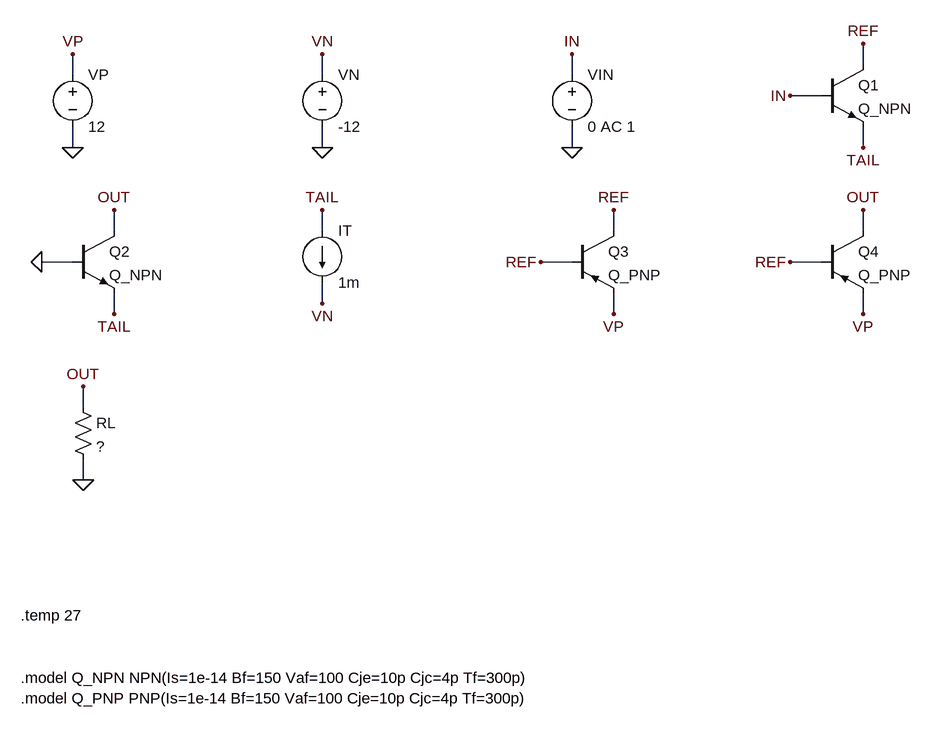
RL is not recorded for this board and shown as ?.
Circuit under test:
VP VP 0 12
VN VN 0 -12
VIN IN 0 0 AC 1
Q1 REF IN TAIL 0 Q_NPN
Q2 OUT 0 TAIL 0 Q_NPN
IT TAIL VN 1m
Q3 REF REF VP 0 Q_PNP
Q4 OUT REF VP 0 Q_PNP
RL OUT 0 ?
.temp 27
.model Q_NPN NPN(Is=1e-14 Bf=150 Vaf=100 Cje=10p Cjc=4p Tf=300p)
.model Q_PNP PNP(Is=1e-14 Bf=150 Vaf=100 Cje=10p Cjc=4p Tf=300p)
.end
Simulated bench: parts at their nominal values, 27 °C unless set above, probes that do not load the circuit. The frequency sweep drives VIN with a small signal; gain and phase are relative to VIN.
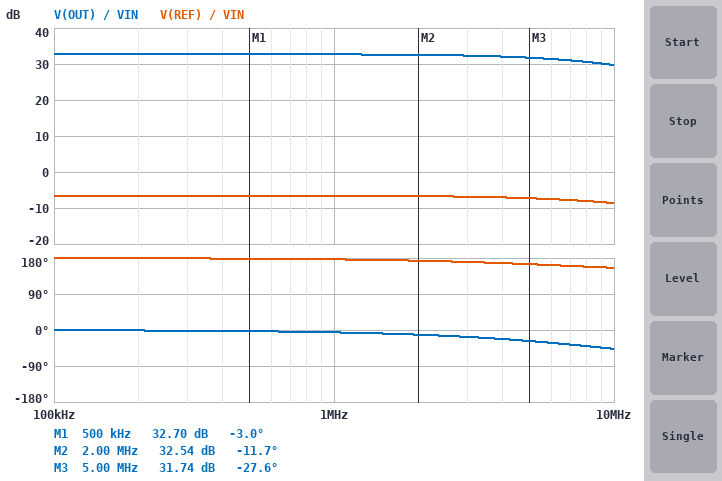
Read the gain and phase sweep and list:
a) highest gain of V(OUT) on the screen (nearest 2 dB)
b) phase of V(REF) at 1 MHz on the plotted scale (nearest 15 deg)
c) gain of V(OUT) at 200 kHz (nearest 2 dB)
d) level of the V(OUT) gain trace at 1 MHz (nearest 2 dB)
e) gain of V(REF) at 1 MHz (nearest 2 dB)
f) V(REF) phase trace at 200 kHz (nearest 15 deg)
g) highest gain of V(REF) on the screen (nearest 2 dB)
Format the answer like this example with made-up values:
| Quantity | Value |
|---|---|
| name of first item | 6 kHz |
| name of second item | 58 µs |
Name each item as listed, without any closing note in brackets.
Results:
| Quantity | Value |
|---|---|
| highest gain of V(OUT) on the screen | 32 dB |
| phase of V(REF) at 1 MHz on the plotted scale | 180 deg |
| gain of V(OUT) at 200 kHz | 32 dB |
| level of the V(OUT) gain trace at 1 MHz | 32 dB |
| gain of V(REF) at 1 MHz | -6 dB |
| V(REF) phase trace at 200 kHz | 180 deg |
| highest gain of V(REF) on the screen | -6 dB |
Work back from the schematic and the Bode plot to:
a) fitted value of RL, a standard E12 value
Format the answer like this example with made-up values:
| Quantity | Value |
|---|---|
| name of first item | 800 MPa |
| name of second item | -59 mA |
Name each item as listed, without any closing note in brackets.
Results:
| Quantity | Value |
|---|---|
| fitted value of RL, a standard E12 value | 2.2 kΩ |
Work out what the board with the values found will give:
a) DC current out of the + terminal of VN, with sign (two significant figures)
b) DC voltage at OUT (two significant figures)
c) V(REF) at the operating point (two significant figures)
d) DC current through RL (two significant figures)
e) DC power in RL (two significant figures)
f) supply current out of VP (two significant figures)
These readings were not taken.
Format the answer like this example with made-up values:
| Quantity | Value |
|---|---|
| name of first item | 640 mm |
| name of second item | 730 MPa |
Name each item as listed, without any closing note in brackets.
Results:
| Quantity | Value |
|---|---|
| DC current out of the + terminal of VN, with sign | -1.0 mA |
| DC voltage at OUT | 230 mV |
| V(REF) at the operating point | 11 V |
| DC current through RL | 100 µA |
| DC power in RL | 23 µW |
| supply current out of VP | 1.1 mA |
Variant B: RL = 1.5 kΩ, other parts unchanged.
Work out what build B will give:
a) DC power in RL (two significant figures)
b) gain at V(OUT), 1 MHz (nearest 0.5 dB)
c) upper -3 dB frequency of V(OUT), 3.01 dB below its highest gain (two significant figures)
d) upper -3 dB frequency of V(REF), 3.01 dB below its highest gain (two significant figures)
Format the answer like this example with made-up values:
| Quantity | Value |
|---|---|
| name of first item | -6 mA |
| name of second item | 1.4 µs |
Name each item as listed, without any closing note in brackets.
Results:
| Quantity | Value |
|---|---|
| DC power in RL | 16 µW |
| gain at V(OUT), 1 MHz | 29.5 dB |
| upper -3 dB frequency of V(OUT), 3.01 dB below its highest gain | 14 MHz |
| upper -3 dB frequency of V(REF), 3.01 dB below its highest gain | 19 MHz |
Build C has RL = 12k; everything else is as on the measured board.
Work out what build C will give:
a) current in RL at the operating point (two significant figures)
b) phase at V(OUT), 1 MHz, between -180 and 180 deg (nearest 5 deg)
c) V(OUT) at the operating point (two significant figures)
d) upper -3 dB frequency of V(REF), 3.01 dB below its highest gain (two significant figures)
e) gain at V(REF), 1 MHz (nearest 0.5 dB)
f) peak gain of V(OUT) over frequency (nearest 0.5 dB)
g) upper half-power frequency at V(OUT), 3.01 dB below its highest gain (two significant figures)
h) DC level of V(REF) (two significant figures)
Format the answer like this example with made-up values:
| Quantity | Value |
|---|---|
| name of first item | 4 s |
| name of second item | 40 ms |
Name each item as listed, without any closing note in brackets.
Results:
| Quantity | Value |
|---|---|
| current in RL at the operating point | 94 µA |
| phase at V(OUT), 1 MHz, between -180 and 180 deg | -25 deg |
| V(OUT) at the operating point | 1.1 V |
| upper -3 dB frequency of V(REF), 3.01 dB below its highest gain | 3.2 MHz |
| gain at V(REF), 1 MHz | -7.5 dB |
| peak gain of V(OUT) over frequency | 46.5 dB |
| upper half-power frequency at V(OUT), 3.01 dB below its highest gain | 2.3 MHz |
| DC level of V(REF) | 11 V |
